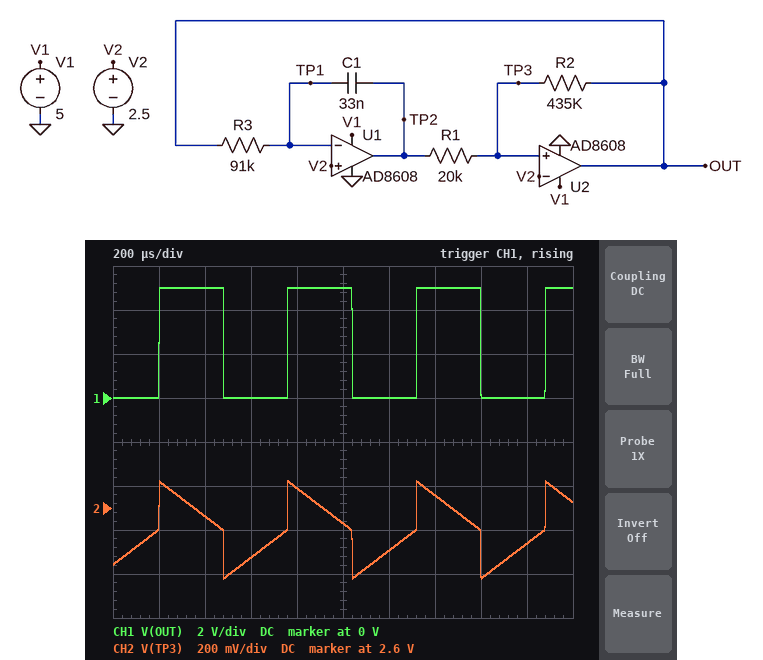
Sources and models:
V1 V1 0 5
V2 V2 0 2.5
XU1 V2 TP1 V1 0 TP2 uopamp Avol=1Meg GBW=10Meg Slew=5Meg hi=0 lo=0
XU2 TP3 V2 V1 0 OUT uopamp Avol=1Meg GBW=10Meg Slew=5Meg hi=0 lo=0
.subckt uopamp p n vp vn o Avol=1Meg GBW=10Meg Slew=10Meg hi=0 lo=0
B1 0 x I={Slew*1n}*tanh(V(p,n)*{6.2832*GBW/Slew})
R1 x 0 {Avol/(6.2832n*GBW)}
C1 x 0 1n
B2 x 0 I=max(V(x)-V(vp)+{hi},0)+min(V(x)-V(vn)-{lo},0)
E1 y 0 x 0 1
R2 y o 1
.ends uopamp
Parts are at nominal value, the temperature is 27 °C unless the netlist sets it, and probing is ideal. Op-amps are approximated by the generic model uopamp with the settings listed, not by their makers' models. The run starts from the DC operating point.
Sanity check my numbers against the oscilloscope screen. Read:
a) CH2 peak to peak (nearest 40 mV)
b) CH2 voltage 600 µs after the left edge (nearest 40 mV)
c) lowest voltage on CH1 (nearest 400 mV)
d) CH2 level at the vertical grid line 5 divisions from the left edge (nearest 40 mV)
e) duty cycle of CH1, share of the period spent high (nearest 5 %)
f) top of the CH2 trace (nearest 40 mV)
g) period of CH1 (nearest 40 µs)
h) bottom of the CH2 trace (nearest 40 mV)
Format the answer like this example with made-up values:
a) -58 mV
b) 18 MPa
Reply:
a) 440 mV
b) 2.36 V
c) 0 V
d) 2.52 V
e) 50 %
f) 2.72 V
g) 560 µs
h) 2.28 V
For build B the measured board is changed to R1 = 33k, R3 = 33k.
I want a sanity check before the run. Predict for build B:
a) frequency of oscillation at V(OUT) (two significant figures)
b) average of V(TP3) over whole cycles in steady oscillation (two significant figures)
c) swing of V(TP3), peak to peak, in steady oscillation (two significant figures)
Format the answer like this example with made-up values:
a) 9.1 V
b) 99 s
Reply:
a) 3.0 kHz
b) 2.5 V
c) 710 mV
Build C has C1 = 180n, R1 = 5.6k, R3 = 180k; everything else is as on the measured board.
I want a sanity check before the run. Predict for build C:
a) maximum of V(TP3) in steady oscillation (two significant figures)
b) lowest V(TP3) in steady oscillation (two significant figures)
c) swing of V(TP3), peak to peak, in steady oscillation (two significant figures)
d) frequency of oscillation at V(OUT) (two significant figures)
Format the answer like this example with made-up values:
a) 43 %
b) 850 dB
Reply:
a) 2.6 V
b) 2.4 V
c) 130 mV
d) 590 Hz
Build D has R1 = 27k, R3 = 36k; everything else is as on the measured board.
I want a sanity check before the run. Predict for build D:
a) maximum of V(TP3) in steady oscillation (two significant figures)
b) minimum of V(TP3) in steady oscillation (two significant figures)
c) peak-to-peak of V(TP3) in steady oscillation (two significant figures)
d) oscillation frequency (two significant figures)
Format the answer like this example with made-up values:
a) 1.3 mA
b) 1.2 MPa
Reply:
a) 2.8 V
b) 2.2 V
c) 590 mV
d) 3.3 kHz
